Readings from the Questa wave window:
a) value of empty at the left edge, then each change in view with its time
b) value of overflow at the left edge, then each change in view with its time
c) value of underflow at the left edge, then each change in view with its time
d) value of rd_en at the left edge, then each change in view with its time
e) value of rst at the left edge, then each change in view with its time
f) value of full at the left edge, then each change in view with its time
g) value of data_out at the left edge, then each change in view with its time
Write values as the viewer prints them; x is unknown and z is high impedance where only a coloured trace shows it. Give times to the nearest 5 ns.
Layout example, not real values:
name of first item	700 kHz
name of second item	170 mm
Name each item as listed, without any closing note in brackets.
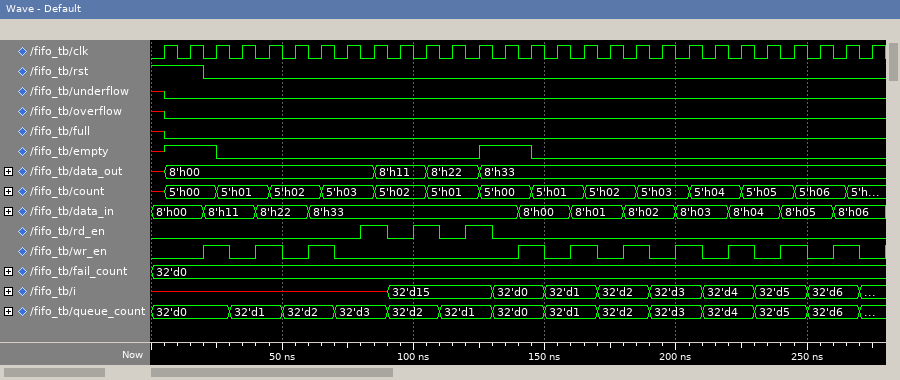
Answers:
value of empty at the left edge, then each change in view with its time	x, 1 at 5 ns, 0 at 25 ns, 1 at 125 ns, 0 at 145 ns
value of overflow at the left edge, then each change in view with its time	x, 0 at 5 ns
value of underflow at the left edge, then each change in view with its time	x, 0 at 5 ns
value of rd_en at the left edge, then each change in view with its time	0, 1 at 80 ns, 0 at 90 ns, 1 at 100 ns, 0 at 110 ns, 1 at 120 ns, 0 at 130 ns
value of rst at the left edge, then each change in view with its time	1, 0 at 20 ns
value of full at the left edge, then each change in view with its time	x, 0 at 5 ns
value of data_out at the left edge, then each change in view with its time	x, 8'h00 at 5 ns, 8'h11 at 85 ns, 8'h22 at 105 ns, 8'h33 at 125 ns
